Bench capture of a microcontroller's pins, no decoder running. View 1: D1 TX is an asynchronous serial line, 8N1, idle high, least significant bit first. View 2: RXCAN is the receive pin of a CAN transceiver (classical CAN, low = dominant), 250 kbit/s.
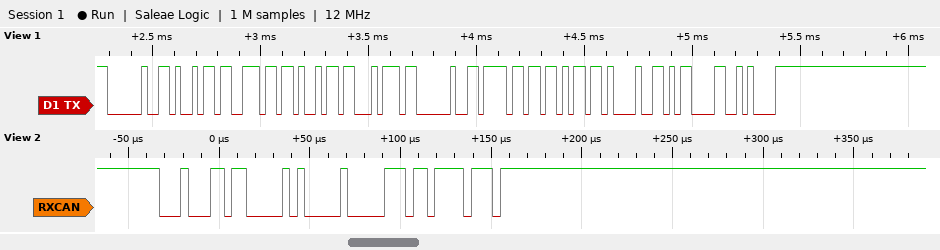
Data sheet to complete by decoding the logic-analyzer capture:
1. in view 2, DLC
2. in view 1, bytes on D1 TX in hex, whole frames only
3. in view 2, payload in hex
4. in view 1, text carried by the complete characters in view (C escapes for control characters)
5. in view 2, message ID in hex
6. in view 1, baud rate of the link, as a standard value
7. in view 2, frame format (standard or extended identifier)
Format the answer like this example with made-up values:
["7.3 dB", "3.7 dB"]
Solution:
["1", "20 69 6E 69 74 20 6F 6B 21 0D 0A", "00", "\" init ok!\\r\\n\"", "0x11B", "38400 baud", "standard"]
